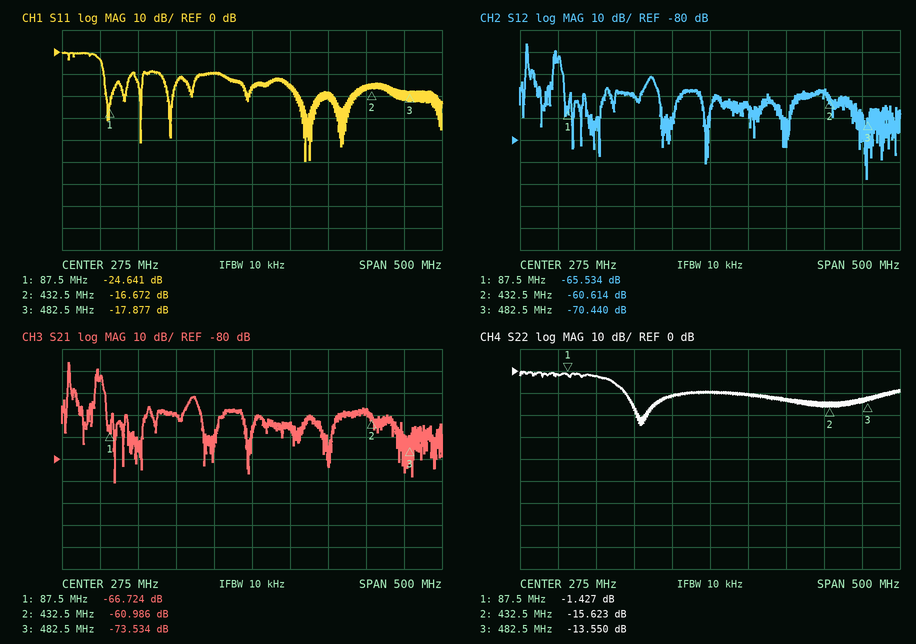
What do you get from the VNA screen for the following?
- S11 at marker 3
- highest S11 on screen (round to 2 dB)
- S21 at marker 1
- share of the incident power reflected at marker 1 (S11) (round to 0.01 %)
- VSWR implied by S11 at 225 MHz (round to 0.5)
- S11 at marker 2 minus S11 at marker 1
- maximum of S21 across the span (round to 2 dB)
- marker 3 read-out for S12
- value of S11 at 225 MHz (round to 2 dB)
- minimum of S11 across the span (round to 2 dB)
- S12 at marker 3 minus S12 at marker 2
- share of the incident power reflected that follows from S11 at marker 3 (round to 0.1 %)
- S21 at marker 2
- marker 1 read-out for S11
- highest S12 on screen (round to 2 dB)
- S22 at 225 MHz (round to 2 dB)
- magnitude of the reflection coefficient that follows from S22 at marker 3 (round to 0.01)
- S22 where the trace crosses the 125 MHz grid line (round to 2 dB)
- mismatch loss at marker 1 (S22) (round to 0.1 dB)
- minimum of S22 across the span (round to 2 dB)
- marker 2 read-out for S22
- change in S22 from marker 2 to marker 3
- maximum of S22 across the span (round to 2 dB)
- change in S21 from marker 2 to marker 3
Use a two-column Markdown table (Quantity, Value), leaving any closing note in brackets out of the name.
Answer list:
| Quantity | Value |
|---|---|
| S11 at marker 3 | -17.877 dB |
| highest S11 on screen | 0 dB |
| S21 at marker 1 | -66.724 dB |
| share of the incident power reflected at marker 1 (S11) | 0.34 % |
| VSWR implied by S11 at 225 MHz | 2.0 |
| S11 at marker 2 minus S11 at marker 1 | 7.969 dB |
| maximum of S21 across the span | -36 dB |
| marker 3 read-out for S12 | -70.440 dB |
| value of S11 at 225 MHz | -10 dB |
| minimum of S11 across the span | -50 dB |
| S12 at marker 3 minus S12 at marker 2 | -9.826 dB |
| share of the incident power reflected that follows from S11 at marker 3 | 1.6 % |
| S21 at marker 2 | -60.986 dB |
| marker 1 read-out for S11 | -24.641 dB |
| highest S12 on screen | -36 dB |
| S22 at 225 MHz | -12 dB |
| magnitude of the reflection coefficient that follows from S22 at marker 3 | 0.21 |
| S22 where the trace crosses the 125 MHz grid line | -2 dB |
| mismatch loss at marker 1 (S22) | 5.5 dB |
| minimum of S22 across the span | -24 dB |
| marker 2 read-out for S22 | -15.623 dB |
| change in S22 from marker 2 to marker 3 | 2.073 dB |
| maximum of S22 across the span | 0 dB |
| change in S21 from marker 2 to marker 3 | -12.548 dB |
